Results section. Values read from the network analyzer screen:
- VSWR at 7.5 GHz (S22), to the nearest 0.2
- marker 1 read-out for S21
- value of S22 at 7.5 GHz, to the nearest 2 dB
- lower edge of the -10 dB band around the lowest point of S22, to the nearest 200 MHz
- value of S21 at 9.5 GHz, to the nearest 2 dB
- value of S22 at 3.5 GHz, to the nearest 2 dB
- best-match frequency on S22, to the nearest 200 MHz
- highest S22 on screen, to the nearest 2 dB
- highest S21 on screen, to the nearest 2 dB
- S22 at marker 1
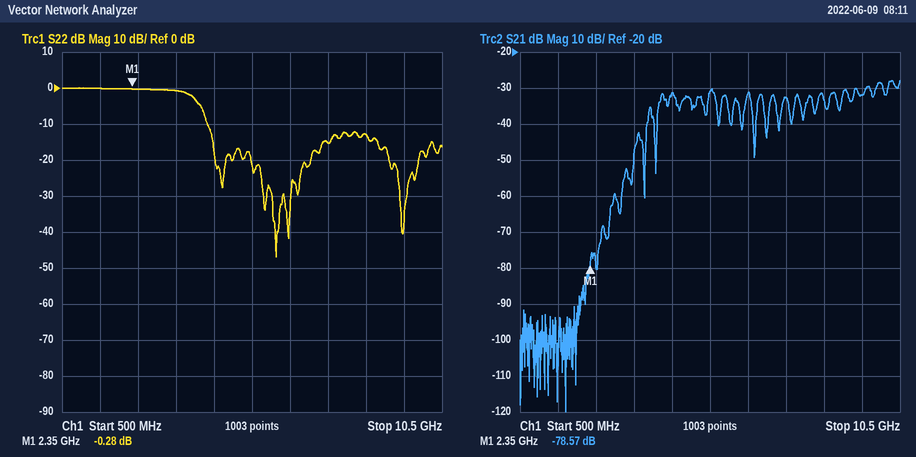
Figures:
1.4
-78.57 dB
-16 dB
4.4 GHz
-32 dB
0 dB
6.2 GHz
0 dB
-28 dB
-0.28 dB
